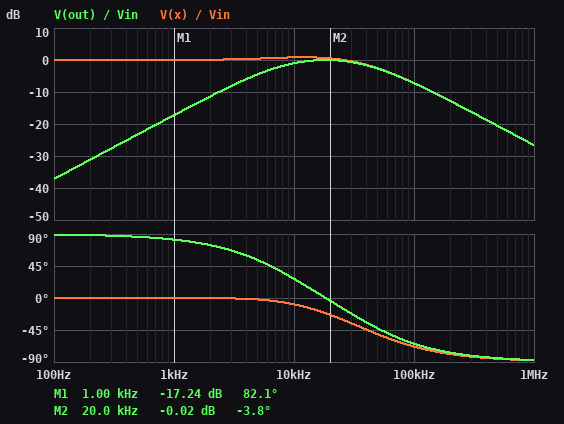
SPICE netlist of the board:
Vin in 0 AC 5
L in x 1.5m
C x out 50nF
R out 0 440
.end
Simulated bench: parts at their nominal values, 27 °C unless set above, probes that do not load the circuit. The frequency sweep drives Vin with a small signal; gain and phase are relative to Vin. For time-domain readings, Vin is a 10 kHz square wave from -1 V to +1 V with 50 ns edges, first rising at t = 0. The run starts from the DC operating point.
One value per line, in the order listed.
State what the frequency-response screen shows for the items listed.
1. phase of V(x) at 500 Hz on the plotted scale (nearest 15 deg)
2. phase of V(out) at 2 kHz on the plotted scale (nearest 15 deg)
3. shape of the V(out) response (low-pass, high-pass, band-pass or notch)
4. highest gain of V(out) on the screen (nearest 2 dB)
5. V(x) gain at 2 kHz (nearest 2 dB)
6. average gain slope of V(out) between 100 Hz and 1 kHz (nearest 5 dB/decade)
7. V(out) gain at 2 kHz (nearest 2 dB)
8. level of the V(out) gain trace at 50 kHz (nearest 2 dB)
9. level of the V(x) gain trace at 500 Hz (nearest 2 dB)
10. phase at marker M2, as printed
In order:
0 deg
75 deg
band-pass
0 dB
0 dB
20 dB/decade
-12 dB
-2 dB
0 dB
-3.8 deg
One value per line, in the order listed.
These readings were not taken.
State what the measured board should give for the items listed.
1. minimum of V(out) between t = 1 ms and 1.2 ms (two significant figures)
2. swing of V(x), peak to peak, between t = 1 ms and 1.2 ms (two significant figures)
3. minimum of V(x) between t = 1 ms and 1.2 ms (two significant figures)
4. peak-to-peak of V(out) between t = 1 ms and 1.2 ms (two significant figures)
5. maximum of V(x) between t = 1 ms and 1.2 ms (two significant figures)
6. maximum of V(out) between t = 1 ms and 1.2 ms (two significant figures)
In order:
-1.5 V
2.4 V
-1.2 V
2.9 V
1.2 V
1.5 V
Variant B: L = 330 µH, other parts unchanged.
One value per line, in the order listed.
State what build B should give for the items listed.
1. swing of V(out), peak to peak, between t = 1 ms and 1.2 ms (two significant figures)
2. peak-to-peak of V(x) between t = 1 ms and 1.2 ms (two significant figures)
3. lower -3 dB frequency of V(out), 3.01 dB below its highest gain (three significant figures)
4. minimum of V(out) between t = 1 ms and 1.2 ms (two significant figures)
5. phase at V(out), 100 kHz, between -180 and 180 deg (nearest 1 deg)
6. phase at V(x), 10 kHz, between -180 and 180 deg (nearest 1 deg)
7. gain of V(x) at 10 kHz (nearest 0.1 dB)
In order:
3.3 V
2.1 V
7.00 kHz
-1.7 V
-22 deg
-2 deg
0.2 dB
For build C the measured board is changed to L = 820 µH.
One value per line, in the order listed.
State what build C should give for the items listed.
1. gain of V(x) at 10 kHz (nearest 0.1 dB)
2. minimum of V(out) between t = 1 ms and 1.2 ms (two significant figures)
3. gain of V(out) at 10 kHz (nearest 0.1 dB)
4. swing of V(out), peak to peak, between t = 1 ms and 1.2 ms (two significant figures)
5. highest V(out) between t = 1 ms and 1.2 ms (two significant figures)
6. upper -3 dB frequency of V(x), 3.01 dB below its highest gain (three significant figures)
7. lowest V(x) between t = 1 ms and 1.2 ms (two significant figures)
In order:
0.5 dB
-1.6 V
-1.4 dB
3.1 V
1.6 V
83.2 kHz
-1.1 V
